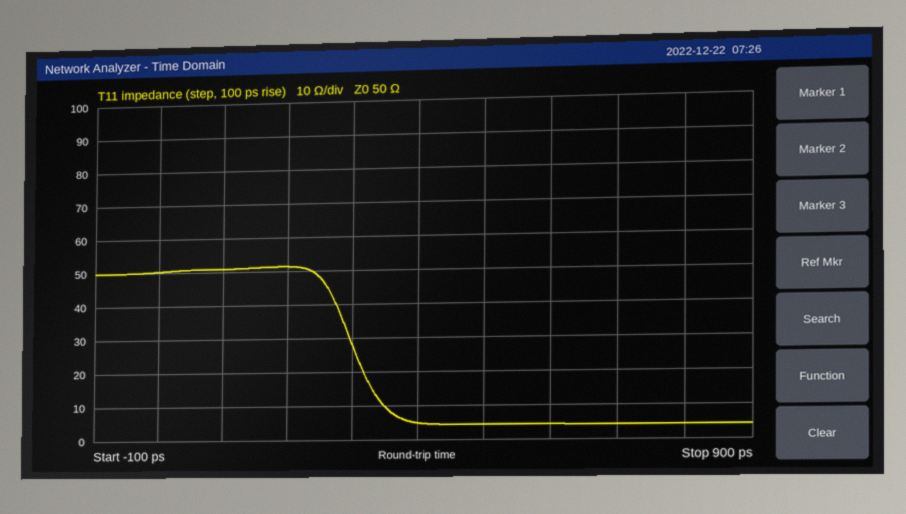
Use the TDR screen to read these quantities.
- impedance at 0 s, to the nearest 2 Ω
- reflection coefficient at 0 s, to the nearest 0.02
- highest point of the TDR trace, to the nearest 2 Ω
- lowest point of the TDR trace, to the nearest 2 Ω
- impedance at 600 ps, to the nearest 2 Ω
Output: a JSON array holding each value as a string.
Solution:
["50 Ω", "0.00", "52 Ω", "4 Ω", "4 Ω"]
